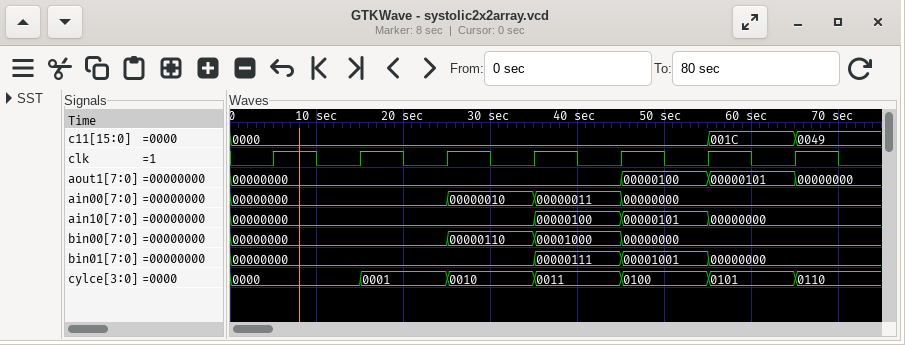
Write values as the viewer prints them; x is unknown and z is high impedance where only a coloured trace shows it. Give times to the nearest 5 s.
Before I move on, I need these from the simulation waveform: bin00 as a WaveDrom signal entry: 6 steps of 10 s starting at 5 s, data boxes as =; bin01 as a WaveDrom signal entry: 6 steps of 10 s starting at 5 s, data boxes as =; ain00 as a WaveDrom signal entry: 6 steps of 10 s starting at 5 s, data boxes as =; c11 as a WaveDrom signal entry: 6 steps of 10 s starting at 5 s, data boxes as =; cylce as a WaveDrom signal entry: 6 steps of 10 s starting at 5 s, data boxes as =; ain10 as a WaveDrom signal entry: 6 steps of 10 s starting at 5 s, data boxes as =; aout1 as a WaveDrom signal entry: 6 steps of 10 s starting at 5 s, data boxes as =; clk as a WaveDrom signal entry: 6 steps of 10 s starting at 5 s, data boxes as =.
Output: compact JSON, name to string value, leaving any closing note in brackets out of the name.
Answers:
{"bin00 as a WaveDrom signal entry: 6 steps of 10 s starting at 5 s, data boxes as =": "{name: 'bin00', wave: '=.===.', data: '00000000 00000110 00001000 00000000'}", "bin01 as a WaveDrom signal entry: 6 steps of 10 s starting at 5 s, data boxes as =": "{name: 'bin01', wave: '=..===', data: '00000000 00000111 00001001 00000000'}", "ain00 as a WaveDrom signal entry: 6 steps of 10 s starting at 5 s, data boxes as =": "{name: 'ain00', wave: '=.===.', data: '00000000 00000010 00000011 00000000'}", "c11 as a WaveDrom signal entry: 6 steps of 10 s starting at 5 s, data boxes as =": "{name: 'c11', wave: '=....=', data: '0000 001C'}", "cylce as a WaveDrom signal entry: 6 steps of 10 s starting at 5 s, data boxes as =": "{name: 'cylce', wave: '======', data: '0000 0001 0010 0011 0100 0101'}", "ain10 as a WaveDrom signal entry: 6 steps of 10 s starting at 5 s, data boxes as =": "{name: 'ain10', wave: '=..===', data: '00000000 00000100 00000101 00000000'}", "aout1 as a WaveDrom signal entry: 6 steps of 10 s starting at 5 s, data boxes as =": "{name: 'aout1', wave: '=...==', data: '00000000 00000100 00000101'}", "clk as a WaveDrom signal entry: 6 steps of 10 s starting at 5 s, data boxes as =": "{name: 'clk', wave: 'p.....'}"}
